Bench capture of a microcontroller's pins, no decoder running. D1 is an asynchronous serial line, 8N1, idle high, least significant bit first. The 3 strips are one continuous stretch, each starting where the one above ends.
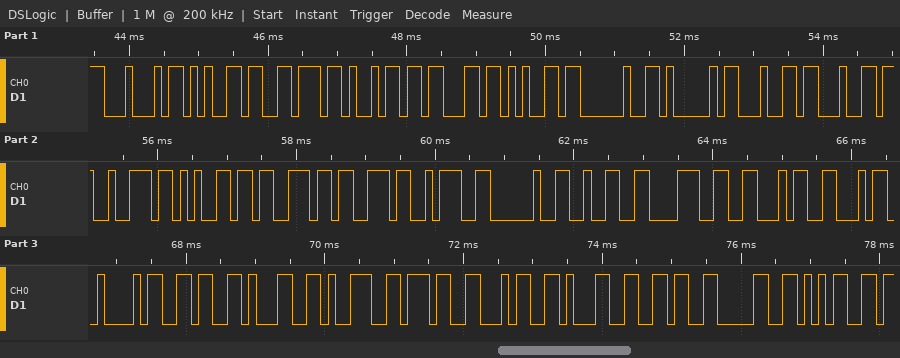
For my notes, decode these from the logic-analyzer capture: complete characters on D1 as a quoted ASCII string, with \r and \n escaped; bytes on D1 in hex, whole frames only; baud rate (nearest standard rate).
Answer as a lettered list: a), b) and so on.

a) "Device Address: 28FFB619741605"
b) 0x44 0x65 0x76 0x69 0x63 0x65 0x20 0x41 0x64 0x64 0x72 0x65 0x73 0x73 0x3A 0x20 0x32 0x38 0x46 0x46 0x42 0x36 0x31 0x39 0x37 0x34 0x31 0x36 0x30 0x35
c) 9600 baud
